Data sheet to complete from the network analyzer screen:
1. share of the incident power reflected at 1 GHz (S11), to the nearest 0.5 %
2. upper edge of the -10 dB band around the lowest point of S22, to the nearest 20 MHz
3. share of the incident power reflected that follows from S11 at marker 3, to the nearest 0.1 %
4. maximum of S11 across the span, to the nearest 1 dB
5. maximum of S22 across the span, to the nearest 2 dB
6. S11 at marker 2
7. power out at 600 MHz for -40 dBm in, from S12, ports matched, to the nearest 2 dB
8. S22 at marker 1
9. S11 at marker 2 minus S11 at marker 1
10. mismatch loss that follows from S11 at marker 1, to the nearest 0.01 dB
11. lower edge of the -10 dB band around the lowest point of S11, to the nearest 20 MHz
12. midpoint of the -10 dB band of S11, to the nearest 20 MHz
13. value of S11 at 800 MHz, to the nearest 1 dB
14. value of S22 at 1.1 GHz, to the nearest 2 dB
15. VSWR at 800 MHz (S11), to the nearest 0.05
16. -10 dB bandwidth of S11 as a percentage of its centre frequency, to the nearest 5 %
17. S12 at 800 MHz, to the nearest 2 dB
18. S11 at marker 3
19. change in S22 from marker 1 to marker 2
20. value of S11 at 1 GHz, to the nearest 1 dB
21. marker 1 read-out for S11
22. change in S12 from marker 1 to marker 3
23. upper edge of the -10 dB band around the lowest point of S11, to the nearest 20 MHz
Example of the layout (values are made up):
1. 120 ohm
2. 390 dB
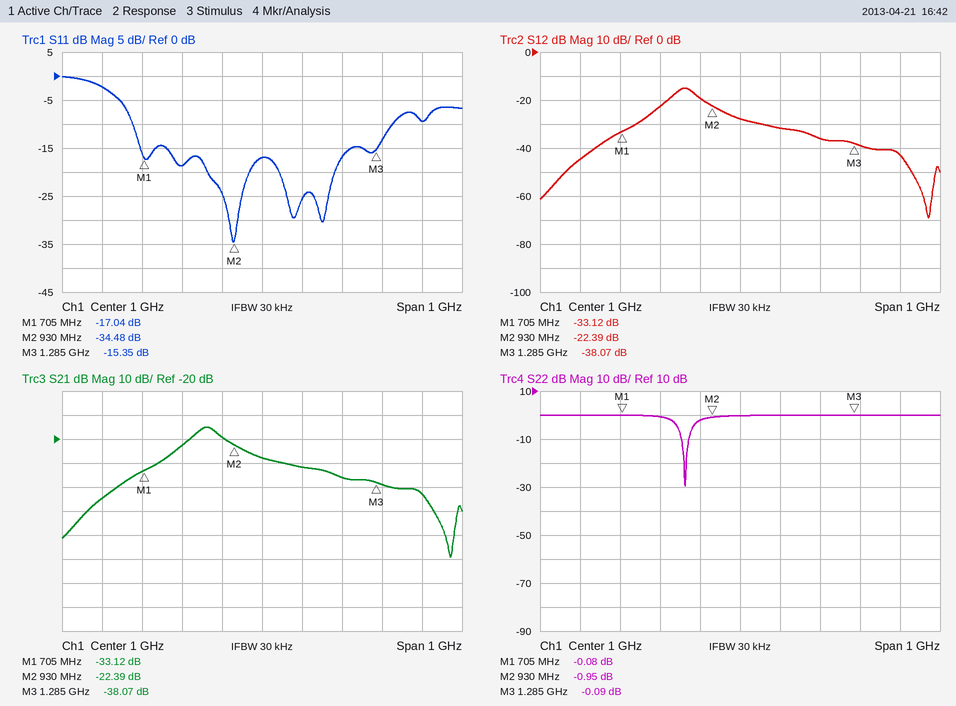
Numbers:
1. 2.0 %
2. 880 MHz
3. 2.9 %
4. 0 dB
5. 0 dB
6. -34.48 dB
7. -84 dBm
8. -0.08 dB
9. -17.44 dB
10. 0.09 dB
11. 680 MHz
12. 1.00 GHz
13. -19 dB
14. 0 dB
15. 1.25
16. 65 %
17. -22 dB
18. -15.35 dB
19. -0.87 dB
20. -17 dB
21. -17.04 dB
22. -4.95 dB
23. 1.32 GHz
